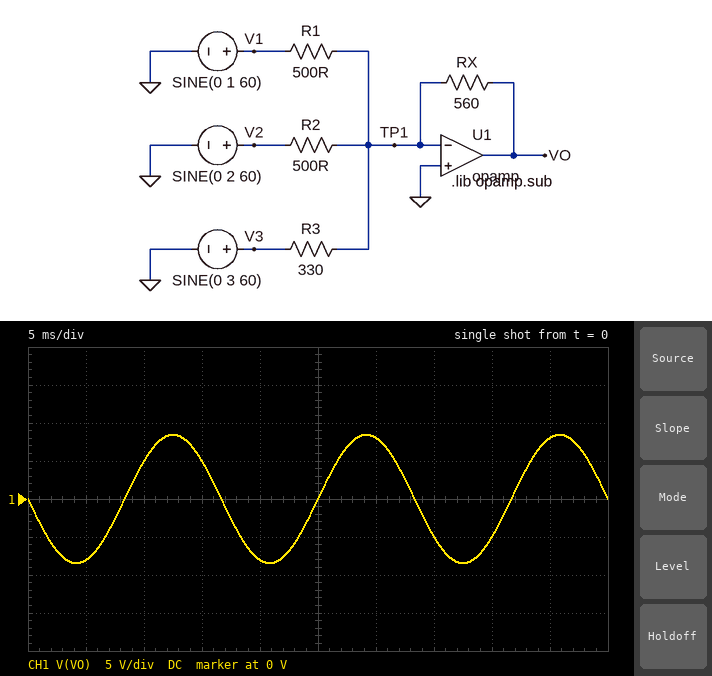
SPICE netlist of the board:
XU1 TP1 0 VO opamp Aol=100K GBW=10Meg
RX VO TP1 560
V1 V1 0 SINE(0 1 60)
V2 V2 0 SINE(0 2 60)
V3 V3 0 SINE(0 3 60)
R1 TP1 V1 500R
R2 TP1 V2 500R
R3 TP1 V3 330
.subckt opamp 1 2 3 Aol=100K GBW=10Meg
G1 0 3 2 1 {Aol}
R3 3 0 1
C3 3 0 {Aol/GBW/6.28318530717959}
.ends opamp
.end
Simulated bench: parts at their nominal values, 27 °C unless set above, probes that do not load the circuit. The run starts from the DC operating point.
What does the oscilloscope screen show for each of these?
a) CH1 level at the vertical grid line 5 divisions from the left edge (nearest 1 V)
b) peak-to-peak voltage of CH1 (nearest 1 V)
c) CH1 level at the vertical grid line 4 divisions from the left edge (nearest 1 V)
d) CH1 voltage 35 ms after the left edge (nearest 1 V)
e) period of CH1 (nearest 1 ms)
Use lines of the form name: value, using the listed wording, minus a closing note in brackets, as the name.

CH1 level at the vertical grid line 5 divisions from the left edge: 0 V
peak-to-peak voltage of CH1: 17 V
CH1 level at the vertical grid line 4 divisions from the left edge: -8 V
CH1 voltage 35 ms after the left edge: -5 V
period of CH1: 17 ms
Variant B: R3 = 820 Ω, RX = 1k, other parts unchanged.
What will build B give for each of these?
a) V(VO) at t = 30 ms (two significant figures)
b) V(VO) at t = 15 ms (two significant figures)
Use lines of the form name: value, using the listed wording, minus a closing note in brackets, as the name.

V(VO) at t = 30 ms: 9.2 V
V(VO) at t = 15 ms: 5.7 V
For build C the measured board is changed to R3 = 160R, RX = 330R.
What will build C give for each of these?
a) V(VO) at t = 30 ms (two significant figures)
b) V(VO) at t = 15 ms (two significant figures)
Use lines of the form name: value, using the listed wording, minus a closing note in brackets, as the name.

V(VO) at t = 30 ms: 7.8 V
V(VO) at t = 15 ms: 4.8 V
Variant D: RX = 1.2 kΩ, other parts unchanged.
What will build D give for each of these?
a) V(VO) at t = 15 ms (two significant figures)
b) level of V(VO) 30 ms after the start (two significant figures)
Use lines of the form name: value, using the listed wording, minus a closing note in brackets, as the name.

V(VO) at t = 15 ms: 11 V
level of V(VO) 30 ms after the start: 17 V
